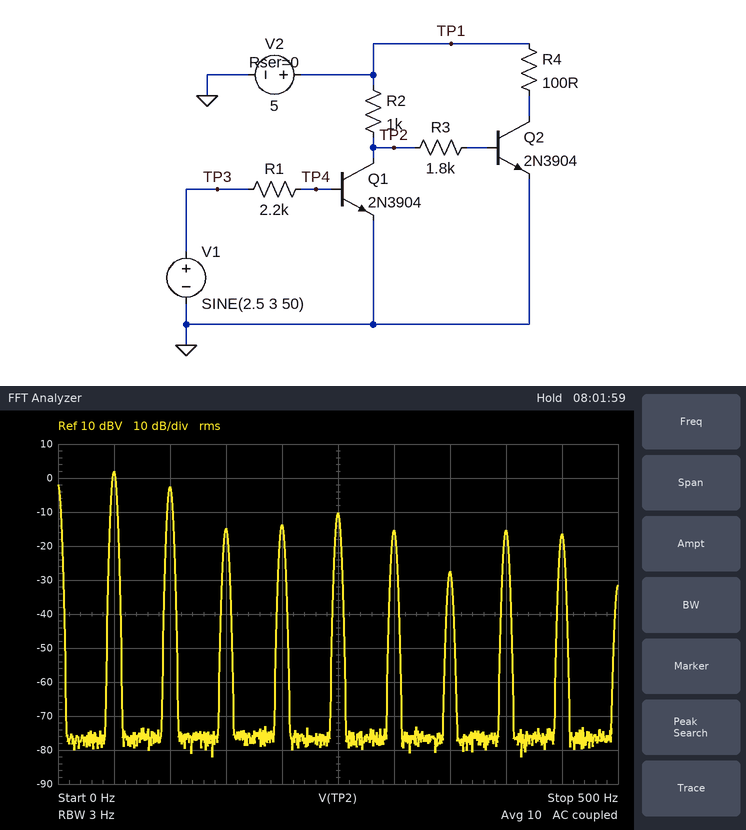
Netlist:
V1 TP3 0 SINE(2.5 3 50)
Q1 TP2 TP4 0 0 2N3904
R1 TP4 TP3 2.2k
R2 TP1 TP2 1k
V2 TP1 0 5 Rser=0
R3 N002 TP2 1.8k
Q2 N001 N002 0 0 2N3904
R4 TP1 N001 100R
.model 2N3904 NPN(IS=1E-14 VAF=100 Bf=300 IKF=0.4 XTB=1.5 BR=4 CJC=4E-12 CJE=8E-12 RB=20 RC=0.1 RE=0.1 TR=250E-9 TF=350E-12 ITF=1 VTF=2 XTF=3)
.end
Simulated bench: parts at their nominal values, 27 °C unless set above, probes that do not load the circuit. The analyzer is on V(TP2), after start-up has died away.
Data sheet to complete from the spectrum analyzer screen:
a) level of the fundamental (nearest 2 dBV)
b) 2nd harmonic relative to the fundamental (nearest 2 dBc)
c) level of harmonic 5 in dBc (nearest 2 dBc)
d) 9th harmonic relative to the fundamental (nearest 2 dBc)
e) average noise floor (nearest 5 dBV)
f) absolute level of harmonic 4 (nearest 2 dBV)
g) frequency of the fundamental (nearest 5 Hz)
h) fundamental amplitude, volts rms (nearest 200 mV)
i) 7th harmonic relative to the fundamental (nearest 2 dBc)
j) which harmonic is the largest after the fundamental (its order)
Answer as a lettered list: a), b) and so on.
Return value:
a) 2 dBV
b) -4 dBc
c) -12 dBc
d) -18 dBc
e) -75 dBV
f) -14 dBV
g) 50 Hz
h) 1.2 V
i) -30 dBc
j) 2
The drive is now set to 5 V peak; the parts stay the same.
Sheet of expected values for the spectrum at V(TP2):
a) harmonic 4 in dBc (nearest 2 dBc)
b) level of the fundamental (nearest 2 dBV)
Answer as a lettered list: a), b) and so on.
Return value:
a) -12 dBc
b) 4 dBV
